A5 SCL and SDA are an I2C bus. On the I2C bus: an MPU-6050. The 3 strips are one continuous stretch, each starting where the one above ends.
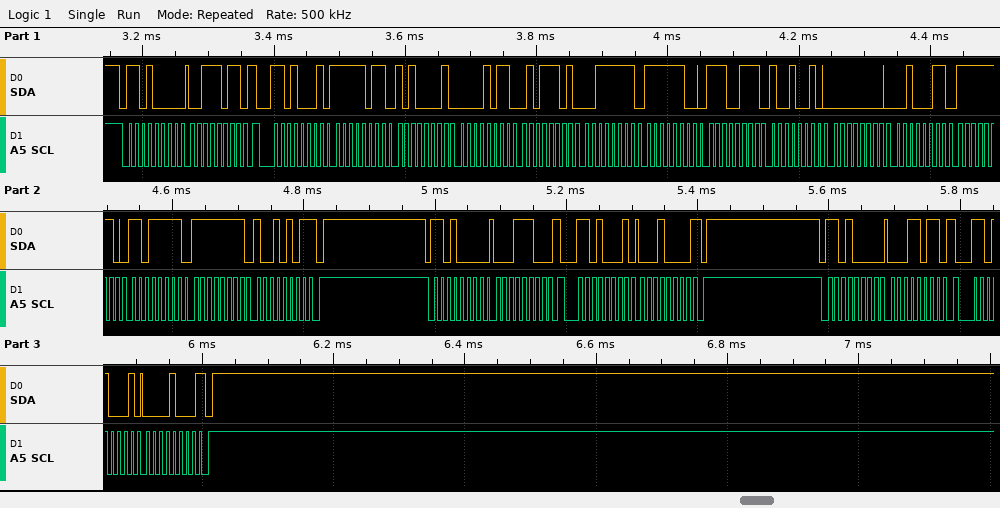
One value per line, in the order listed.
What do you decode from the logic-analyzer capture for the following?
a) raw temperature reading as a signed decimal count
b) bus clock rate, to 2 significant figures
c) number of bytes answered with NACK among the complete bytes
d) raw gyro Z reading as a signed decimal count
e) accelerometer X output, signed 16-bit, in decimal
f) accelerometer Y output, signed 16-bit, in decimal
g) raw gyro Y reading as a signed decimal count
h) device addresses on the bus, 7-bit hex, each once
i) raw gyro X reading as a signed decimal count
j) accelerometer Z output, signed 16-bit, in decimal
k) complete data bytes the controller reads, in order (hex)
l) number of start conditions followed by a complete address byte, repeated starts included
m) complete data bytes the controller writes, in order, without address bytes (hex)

-6254
100 kHz
3
-107
-1119
2909
-289
0x68
35
16380
FB A1 0B 5D 3F FC E7 92 00 23 FE DF FF 95 10 08
6
3B 1C 1B
